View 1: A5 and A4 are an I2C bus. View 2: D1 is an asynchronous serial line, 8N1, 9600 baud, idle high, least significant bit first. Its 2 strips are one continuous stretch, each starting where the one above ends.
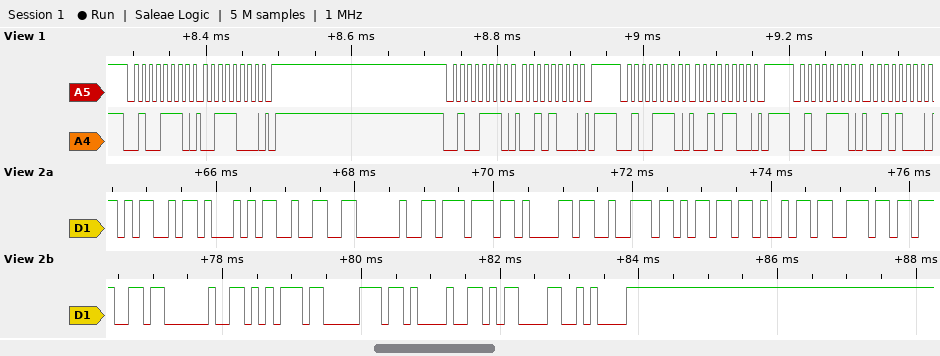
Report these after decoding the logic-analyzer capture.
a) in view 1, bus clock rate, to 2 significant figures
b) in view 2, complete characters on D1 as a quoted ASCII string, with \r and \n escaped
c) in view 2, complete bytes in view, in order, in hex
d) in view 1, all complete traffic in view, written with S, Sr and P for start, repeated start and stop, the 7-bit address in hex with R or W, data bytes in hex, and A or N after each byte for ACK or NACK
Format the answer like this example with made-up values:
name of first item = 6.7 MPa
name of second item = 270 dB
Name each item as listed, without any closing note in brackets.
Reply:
in view 1, bus clock rate, to 2 significant figures = 100 kHz
in view 2, complete characters on D1 as a quoted ASCII string, with \r and \n escaped = "MQ2 warming up!\r\n"
in view 2, complete bytes in view, in order, in hex = 0x4D 0x51 0x32 0x20 0x77 0x61 0x72 0x6D 0x69 0x6E 0x67 0x20 0x75 0x70 0x21 0x0D 0x0A
in view 1, all complete traffic in view, written with S, Sr and P for start, repeated start and stop, the 7-bit address in hex with R or W, data bytes in hex, and A or N after each byte for ACK or NACK = S 27W A 38 A P S 27W A 28 A P S 27W A 2C A P S 27W A 28 A
